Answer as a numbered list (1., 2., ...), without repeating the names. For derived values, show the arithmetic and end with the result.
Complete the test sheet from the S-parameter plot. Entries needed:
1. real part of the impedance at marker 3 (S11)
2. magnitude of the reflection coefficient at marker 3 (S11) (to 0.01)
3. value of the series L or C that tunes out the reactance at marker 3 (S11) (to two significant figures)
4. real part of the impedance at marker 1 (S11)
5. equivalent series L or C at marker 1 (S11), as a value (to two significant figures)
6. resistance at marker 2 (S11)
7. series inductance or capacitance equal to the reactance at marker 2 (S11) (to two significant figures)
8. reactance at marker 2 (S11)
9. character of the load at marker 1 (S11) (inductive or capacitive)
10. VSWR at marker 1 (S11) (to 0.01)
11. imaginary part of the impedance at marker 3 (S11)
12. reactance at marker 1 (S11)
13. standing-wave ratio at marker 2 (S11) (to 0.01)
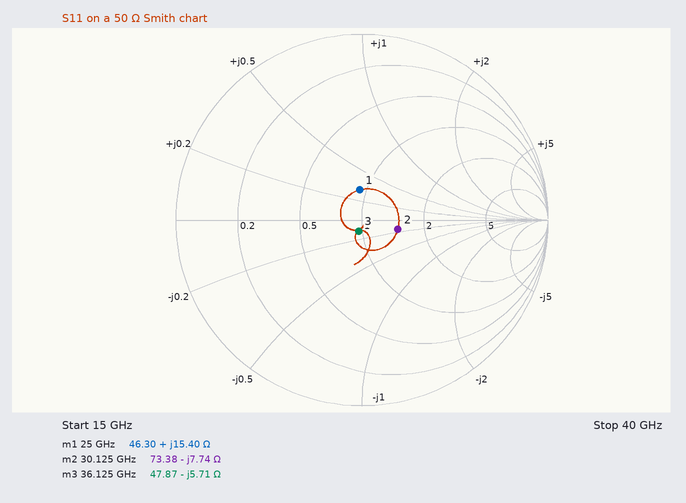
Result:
1. 47.87 Ω
2. 0.06
3. L = 5.71 Ω/(2π × 36.125 GHz) ≈ 25 pH
4. 46.30 Ω
5. L = 15.4 Ω/(2π × 25 GHz) ≈ 98 pH
6. 73.38 Ω
7. C = 1/(2π × 30.125 GHz × 7.74 Ω) ≈ 683 fF, so 680 fF to two significant figures
8. -7.74 Ω
9. inductive
10. 1.39
11. -5.71 Ω
12. +15.40 Ω
13. 1.50
